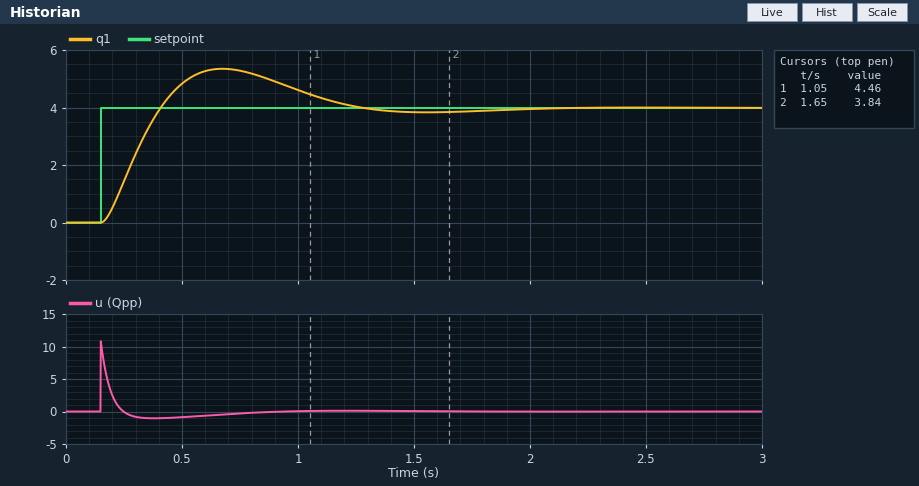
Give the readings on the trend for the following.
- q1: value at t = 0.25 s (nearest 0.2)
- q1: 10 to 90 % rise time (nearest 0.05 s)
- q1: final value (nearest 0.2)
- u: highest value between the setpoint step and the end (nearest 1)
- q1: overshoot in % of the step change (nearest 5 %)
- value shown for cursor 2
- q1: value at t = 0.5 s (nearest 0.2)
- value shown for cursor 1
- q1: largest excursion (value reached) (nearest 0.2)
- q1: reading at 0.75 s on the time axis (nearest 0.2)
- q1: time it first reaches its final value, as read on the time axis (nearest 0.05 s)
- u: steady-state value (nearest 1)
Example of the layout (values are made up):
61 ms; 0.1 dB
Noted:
1.4; 0.20 s; 4.0; 11; 35 %; 3.84; 4.8; 4.46; 5.4; 5.2; 0.40 s; 0
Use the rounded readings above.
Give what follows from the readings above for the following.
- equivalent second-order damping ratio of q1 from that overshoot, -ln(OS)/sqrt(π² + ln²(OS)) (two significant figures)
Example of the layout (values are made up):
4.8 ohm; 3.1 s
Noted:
0.32
